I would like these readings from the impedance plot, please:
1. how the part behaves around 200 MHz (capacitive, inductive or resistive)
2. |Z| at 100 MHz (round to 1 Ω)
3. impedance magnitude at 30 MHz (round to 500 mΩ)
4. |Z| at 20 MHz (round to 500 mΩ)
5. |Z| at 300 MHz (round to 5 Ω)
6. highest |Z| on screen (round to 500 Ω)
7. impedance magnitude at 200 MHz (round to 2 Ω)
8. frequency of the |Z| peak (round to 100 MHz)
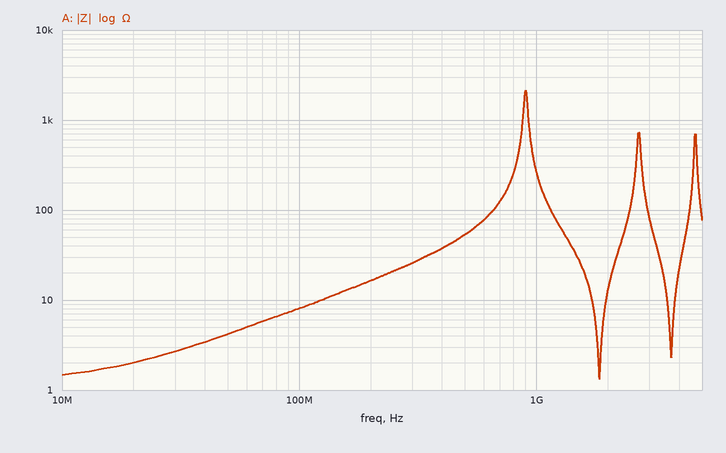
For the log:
inductive
8 Ω
2.5 Ω
2.0 Ω
25 Ω
2.0 kΩ
16 Ω
900 MHz
